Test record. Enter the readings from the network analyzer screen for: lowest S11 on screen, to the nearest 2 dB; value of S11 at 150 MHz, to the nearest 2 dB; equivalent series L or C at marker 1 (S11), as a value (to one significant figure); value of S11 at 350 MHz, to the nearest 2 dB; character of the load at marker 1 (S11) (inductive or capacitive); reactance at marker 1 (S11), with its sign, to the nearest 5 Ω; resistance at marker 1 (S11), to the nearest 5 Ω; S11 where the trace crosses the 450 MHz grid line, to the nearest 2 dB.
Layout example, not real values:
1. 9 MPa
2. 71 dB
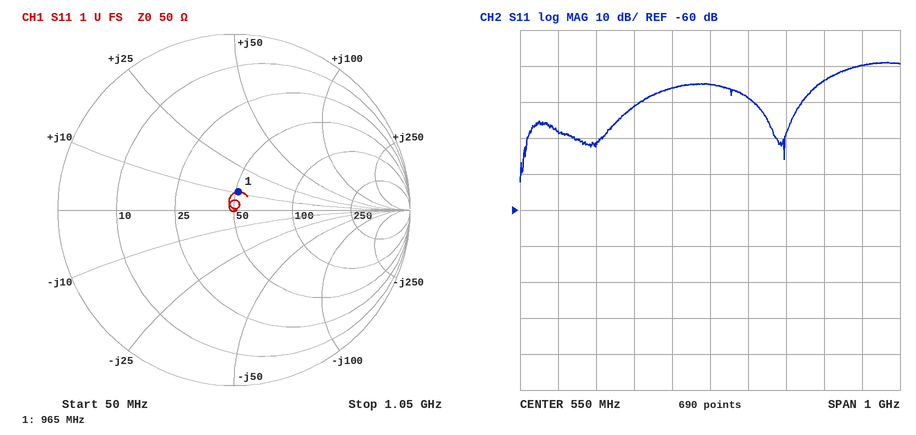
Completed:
1. -52 dB
2. -38 dB
3. 2 nH
4. -32 dB
5. inductive
6. +10 Ω
7. 50 Ω
8. -26 dB
